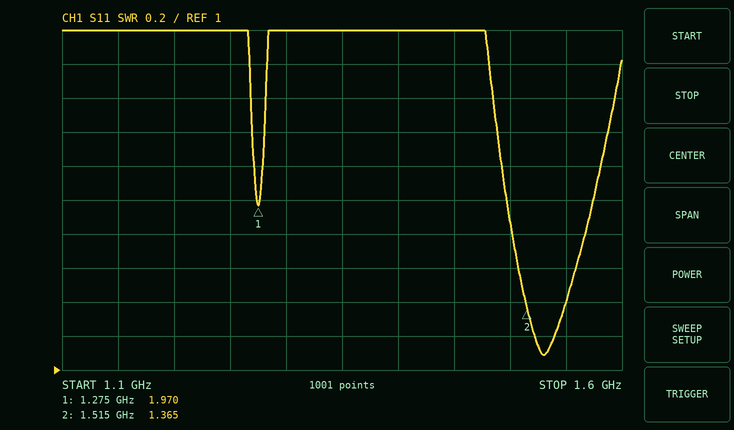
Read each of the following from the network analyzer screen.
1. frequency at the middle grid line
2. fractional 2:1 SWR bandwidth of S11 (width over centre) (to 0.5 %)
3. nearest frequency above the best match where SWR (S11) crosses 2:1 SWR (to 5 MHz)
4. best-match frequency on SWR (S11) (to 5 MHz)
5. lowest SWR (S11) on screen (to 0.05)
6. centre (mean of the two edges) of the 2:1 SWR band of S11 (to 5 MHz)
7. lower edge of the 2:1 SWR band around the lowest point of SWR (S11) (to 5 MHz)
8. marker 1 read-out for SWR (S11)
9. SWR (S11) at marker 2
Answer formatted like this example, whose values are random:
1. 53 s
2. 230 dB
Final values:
1. 1.35 GHz
2. 5.0 %
3. 1.575 GHz
4. 1.530 GHz
5. 1.10
6. 1.535 GHz
7. 1.495 GHz
8. 1.970
9. 1.365
